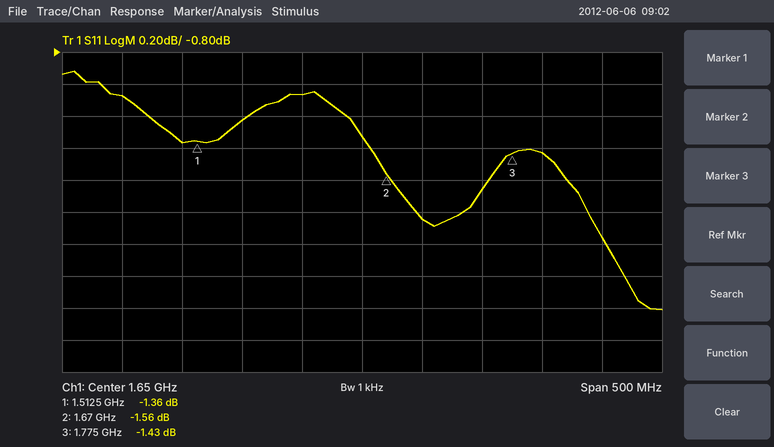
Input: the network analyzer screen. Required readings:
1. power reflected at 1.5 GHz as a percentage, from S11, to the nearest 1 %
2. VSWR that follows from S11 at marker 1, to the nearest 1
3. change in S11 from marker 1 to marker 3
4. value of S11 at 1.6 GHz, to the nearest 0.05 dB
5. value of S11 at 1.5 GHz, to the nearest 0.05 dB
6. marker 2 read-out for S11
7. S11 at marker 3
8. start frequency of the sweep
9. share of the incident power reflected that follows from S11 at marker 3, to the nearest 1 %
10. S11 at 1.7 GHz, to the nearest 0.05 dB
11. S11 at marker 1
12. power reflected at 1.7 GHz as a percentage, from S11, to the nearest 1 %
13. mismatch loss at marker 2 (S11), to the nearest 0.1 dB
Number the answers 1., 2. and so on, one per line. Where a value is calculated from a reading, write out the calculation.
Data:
1. 10^(-1.35/10) ≈ 73 %
2. (1 + 0.8551)/(1 − 0.8551) ≈ 13
3. -1.43 − (-1.36) = -0.07 dB
4. -1.05 dB
5. -1.35 dB
6. -1.56 dB
7. -1.43 dB
8. 1.4 GHz
9. 10^(-1.43/10) ≈ 72 %
10. -1.85 dB
11. -1.36 dB
12. 10^(-1.85/10) ≈ 65 %
13. −10 log10(1 − 10^(-1.56/10)) ≈ 5.2 dB
